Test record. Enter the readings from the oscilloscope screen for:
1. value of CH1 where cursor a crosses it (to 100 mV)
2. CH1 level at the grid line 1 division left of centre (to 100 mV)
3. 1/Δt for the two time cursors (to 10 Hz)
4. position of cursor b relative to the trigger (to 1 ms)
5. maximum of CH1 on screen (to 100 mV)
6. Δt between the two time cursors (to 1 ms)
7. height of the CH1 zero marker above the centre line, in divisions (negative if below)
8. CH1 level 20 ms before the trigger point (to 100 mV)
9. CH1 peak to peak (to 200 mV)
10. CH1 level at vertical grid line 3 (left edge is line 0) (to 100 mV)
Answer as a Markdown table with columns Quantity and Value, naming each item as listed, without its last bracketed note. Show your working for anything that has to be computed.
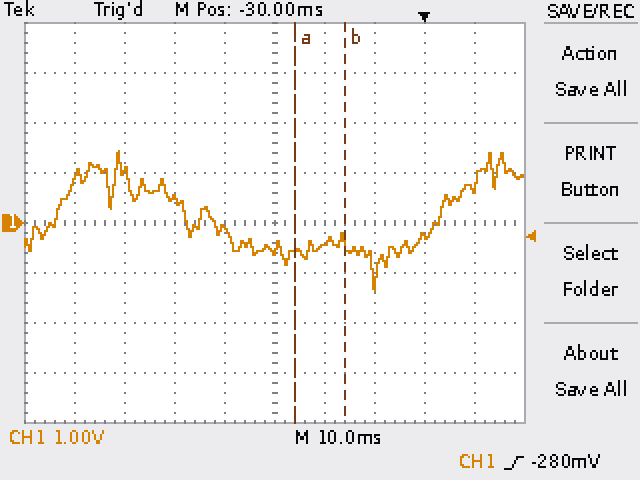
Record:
| Quantity | Value |
|---|---|
| value of CH1 where cursor a crosses it | -600 mV |
| CH1 level at the grid line 1 division left of centre | -100 mV |
| 1/Δt for the two time cursors | 1 / 10 ms ≈ 100 Hz |
| position of cursor b relative to the trigger | -16 ms |
| maximum of CH1 on screen | 1.4 V |
| Δt between the two time cursors | 10 ms |
| height of the CH1 zero marker above the centre line, in divisions | 0.0 div |
| CH1 level 20 ms before the trigger point | -400 mV |
| CH1 peak to peak | 2.8 V |
| CH1 level at vertical grid line 3 (left edge is line 0) | 500 mV |
